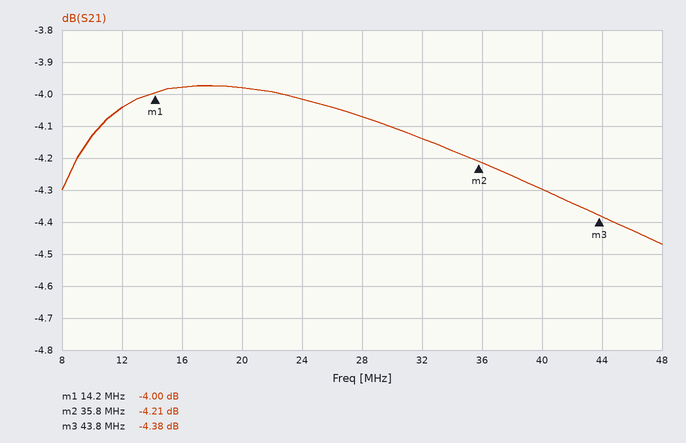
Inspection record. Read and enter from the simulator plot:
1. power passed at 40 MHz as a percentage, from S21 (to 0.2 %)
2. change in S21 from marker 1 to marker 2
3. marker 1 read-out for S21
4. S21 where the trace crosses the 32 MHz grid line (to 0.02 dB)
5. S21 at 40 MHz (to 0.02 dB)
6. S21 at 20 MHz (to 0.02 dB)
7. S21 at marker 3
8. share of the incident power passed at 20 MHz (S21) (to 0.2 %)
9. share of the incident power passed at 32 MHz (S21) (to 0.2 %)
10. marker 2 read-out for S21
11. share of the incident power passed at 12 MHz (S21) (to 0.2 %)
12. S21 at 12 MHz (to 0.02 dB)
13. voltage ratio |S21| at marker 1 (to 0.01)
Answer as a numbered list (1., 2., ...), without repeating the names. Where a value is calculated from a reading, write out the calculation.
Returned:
1. 10^(-4.3/10) ≈ 37.2 %
2. -4.21 − (-4) = -0.21 dB
3. -4.00 dB
4. -4.14 dB
5. -4.30 dB
6. -3.98 dB
7. -4.38 dB
8. 10^(-3.98/10) ≈ 40.0 %
9. 10^(-4.14/10) ≈ 38.5 %, so 38.6 % to the nearest 0.2 %
10. -4.21 dB
11. 10^(-4.04/10) ≈ 39.4 %
12. -4.04 dB
13. 10^(-4/20) ≈ 0.63
